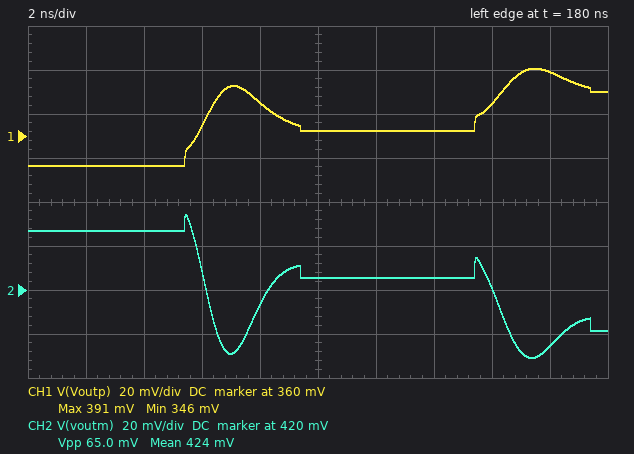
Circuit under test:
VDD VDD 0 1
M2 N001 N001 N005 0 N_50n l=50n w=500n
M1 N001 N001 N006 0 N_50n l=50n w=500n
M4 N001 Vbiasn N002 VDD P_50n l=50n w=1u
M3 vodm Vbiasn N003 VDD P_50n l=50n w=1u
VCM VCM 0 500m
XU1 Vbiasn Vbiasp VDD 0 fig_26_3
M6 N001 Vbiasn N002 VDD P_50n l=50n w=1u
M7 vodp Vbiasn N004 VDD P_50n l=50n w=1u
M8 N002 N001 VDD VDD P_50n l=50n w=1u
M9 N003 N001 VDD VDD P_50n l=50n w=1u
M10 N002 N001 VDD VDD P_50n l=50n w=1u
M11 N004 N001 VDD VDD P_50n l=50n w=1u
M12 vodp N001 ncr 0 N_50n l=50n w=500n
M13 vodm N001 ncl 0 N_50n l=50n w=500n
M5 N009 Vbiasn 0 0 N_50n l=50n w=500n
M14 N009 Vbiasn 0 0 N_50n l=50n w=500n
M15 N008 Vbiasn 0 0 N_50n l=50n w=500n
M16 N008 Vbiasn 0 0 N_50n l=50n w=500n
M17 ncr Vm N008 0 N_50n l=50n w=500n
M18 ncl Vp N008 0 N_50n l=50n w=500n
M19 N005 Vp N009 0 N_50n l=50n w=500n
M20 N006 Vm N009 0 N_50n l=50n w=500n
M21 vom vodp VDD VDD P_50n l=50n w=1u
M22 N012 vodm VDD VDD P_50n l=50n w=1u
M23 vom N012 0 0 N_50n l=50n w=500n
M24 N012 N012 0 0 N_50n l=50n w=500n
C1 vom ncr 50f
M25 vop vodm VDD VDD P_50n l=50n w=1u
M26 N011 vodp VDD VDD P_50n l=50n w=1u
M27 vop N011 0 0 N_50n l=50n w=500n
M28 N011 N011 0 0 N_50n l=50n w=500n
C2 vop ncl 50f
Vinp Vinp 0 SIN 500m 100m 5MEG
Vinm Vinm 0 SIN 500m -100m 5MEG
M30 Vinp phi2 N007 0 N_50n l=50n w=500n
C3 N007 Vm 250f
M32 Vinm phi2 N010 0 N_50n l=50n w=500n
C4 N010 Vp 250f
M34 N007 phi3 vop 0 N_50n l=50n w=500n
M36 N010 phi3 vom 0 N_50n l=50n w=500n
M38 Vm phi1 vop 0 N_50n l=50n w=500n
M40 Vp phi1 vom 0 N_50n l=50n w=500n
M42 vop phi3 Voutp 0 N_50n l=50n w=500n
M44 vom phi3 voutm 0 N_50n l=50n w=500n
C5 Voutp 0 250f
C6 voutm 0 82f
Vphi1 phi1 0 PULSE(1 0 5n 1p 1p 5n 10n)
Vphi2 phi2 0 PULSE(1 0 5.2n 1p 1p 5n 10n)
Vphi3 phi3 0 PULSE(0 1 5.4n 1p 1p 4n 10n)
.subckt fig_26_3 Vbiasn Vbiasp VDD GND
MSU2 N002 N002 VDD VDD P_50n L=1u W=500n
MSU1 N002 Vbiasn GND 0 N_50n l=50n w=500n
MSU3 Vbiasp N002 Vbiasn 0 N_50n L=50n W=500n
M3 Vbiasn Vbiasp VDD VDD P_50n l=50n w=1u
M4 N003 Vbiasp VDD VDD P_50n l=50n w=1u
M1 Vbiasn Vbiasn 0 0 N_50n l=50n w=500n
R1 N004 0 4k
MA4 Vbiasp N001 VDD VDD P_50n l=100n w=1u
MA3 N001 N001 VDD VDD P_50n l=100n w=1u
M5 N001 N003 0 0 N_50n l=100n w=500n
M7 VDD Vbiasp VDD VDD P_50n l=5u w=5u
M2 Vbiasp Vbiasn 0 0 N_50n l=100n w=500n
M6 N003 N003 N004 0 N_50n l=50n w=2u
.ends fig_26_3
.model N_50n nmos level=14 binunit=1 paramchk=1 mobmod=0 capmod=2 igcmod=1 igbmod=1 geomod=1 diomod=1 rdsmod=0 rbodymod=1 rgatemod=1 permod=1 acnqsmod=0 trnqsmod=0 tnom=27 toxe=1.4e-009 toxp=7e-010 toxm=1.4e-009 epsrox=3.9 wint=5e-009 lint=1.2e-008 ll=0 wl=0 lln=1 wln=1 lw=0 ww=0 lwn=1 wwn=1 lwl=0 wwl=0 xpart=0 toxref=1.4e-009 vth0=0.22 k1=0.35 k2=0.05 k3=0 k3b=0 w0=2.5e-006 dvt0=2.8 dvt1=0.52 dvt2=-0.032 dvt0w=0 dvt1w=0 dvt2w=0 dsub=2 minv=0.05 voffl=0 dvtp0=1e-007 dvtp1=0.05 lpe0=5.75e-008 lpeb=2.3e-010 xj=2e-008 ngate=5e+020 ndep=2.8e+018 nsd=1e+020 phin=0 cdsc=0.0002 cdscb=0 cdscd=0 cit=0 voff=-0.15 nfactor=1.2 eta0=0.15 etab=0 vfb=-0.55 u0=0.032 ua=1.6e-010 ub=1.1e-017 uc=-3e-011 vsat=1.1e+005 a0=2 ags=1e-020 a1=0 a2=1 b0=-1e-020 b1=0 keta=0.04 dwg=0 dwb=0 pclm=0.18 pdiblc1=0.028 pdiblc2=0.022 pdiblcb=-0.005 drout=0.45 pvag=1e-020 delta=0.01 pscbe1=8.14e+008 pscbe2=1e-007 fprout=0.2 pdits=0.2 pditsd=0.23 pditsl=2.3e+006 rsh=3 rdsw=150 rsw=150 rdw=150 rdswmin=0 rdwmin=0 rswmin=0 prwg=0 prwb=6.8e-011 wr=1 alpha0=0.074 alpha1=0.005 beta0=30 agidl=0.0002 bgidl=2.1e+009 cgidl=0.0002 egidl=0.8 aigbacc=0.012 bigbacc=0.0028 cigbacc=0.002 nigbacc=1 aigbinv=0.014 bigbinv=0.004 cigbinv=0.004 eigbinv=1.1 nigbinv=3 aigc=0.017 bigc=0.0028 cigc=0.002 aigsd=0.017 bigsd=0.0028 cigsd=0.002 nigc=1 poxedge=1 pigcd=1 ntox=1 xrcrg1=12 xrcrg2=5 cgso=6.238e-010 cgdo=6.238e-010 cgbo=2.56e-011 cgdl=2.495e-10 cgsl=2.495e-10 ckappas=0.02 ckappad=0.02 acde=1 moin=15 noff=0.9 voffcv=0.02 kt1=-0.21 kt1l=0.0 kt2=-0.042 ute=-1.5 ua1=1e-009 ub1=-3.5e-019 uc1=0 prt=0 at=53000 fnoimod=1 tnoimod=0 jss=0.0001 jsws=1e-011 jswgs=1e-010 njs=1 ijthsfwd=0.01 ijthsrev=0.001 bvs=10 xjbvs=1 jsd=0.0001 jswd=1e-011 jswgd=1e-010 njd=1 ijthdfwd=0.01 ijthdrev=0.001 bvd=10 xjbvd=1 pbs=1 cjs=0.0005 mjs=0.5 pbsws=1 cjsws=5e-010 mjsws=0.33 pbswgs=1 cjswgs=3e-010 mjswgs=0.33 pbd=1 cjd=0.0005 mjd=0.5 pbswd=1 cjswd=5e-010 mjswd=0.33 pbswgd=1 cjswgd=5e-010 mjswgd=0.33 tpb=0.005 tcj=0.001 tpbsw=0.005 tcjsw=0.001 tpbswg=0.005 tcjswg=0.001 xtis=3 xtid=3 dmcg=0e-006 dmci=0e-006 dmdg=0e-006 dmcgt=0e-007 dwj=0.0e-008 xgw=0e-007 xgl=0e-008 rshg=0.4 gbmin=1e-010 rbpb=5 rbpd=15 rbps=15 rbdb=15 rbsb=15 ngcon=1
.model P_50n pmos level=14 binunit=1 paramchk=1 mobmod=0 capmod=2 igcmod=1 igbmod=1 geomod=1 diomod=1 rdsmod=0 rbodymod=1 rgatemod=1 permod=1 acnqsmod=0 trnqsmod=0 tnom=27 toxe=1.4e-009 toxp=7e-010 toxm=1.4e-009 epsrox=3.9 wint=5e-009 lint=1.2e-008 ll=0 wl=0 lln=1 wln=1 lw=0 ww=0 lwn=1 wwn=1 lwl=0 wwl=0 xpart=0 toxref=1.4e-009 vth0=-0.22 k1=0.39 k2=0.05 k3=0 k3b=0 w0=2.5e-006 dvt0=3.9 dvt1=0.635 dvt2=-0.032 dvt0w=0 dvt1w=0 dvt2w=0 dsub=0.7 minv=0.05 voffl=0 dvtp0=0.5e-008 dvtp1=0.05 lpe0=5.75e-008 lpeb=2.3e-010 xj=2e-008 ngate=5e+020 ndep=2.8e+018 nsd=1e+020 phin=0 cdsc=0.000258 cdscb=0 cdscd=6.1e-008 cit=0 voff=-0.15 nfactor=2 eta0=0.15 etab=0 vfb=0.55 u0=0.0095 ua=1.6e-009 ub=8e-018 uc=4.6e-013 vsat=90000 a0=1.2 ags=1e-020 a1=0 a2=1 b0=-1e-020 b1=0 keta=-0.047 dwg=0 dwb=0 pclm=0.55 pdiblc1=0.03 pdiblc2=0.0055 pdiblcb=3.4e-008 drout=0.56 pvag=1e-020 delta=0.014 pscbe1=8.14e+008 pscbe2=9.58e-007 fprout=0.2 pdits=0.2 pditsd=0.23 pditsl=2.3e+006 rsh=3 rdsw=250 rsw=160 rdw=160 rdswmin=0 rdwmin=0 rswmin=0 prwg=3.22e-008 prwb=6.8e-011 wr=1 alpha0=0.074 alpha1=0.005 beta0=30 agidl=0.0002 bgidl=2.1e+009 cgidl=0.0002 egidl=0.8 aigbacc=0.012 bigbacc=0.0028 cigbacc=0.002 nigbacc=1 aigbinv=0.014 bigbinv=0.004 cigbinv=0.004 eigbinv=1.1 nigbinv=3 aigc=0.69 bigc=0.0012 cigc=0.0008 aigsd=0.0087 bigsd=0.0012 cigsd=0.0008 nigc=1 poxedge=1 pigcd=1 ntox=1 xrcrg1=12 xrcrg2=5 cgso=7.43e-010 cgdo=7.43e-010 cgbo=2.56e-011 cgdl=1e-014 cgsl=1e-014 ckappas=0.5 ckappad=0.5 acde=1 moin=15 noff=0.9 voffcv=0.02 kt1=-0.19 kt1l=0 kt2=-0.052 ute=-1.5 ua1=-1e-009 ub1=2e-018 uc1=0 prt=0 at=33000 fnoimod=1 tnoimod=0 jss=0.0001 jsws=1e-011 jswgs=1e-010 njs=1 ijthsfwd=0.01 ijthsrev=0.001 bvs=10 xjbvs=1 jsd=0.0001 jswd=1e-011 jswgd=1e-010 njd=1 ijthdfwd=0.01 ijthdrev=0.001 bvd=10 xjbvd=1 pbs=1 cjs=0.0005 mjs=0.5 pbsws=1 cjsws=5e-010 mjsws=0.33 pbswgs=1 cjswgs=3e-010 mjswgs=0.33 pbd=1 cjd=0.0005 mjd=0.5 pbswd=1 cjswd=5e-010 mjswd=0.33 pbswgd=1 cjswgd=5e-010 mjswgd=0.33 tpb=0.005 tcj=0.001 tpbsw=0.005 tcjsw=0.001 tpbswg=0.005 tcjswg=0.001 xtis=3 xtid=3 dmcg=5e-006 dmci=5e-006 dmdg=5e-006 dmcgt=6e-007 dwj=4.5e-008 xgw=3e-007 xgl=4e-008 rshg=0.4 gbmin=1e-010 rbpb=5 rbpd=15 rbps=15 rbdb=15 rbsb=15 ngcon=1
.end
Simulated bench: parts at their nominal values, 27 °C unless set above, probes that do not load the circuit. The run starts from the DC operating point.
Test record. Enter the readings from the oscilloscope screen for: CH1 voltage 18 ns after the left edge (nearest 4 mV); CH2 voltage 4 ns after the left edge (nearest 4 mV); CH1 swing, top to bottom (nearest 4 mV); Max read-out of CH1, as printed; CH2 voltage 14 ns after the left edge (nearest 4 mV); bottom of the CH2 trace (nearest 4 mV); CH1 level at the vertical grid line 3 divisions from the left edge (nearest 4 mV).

388 mV
448 mV
44 mV
391 mV
424 mV
388 mV
364 mV
